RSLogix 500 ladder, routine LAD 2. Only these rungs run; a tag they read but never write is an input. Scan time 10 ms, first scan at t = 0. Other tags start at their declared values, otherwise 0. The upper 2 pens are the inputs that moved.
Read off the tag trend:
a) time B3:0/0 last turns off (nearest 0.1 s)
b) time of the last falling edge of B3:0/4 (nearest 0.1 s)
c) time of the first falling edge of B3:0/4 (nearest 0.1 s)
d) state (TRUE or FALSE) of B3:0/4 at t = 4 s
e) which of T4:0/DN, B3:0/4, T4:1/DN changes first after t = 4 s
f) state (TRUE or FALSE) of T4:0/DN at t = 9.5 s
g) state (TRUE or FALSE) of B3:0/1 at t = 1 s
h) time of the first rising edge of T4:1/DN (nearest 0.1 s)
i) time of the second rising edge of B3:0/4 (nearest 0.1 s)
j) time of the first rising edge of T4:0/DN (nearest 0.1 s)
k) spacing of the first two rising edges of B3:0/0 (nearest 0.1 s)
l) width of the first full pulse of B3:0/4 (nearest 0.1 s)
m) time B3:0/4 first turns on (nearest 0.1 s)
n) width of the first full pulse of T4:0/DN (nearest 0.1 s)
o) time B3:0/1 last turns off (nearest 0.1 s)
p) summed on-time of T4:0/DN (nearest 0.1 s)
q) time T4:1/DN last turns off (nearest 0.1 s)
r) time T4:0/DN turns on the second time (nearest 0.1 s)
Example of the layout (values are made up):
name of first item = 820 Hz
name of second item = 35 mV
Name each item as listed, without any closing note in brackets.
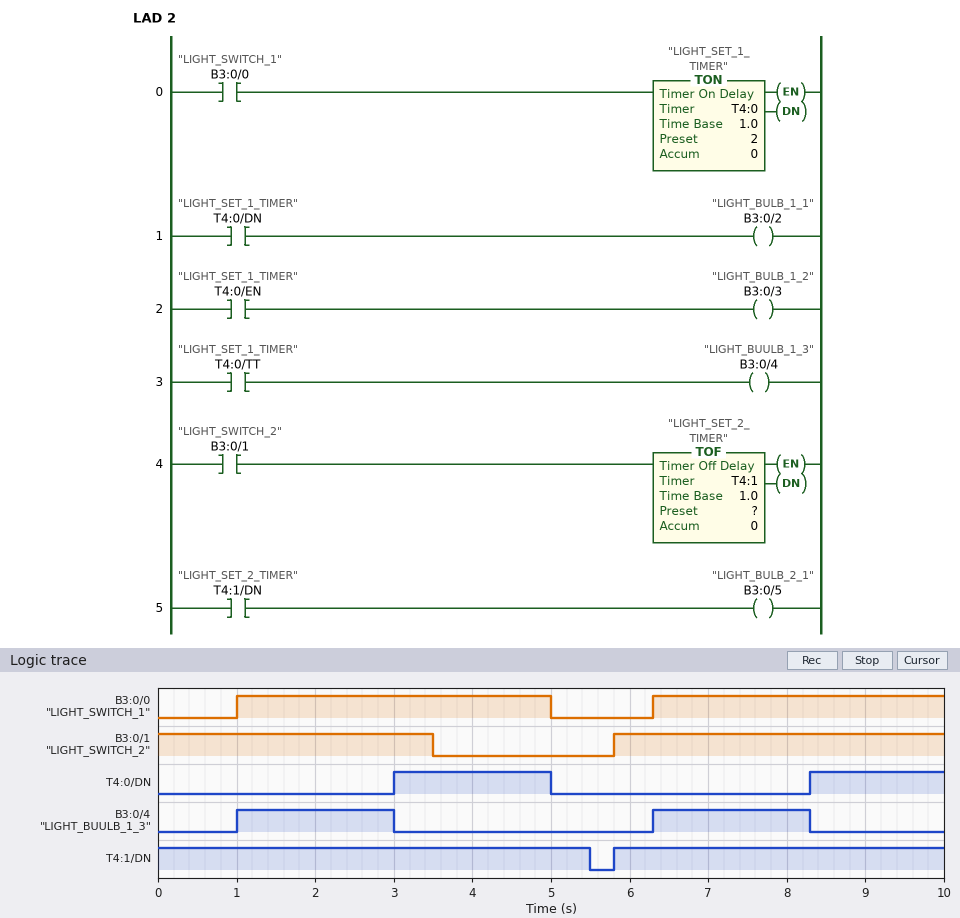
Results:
time B3:0/0 last turns off = 5.0 s
time of the last falling edge of B3:0/4 = 8.3 s
time of the first falling edge of B3:0/4 = 3.0 s
state (TRUE or FALSE) of B3:0/4 at t = 4 s = FALSE
which of T4:0/DN, B3:0/4, T4:1/DN changes first after t = 4 s = T4:0/DN
state (TRUE or FALSE) of T4:0/DN at t = 9.5 s = TRUE
state (TRUE or FALSE) of B3:0/1 at t = 1 s = TRUE
time of the first rising edge of T4:1/DN = 5.8 s
time of the second rising edge of B3:0/4 = 6.3 s
time of the first rising edge of T4:0/DN = 3.0 s
spacing of the first two rising edges of B3:0/0 = 5.3 s
width of the first full pulse of B3:0/4 = 2.0 s
time B3:0/4 first turns on = 1.0 s
width of the first full pulse of T4:0/DN = 2.0 s
time B3:0/1 last turns off = 3.5 s
summed on-time of T4:0/DN = 3.7 s
time T4:1/DN last turns off = 5.5 s
time T4:0/DN turns on the second time = 8.3 s
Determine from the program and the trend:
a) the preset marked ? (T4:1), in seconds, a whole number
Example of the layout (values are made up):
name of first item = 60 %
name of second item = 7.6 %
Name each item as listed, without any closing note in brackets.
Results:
the preset marked ? (T4:1), in seconds, a whole number = 2 s
